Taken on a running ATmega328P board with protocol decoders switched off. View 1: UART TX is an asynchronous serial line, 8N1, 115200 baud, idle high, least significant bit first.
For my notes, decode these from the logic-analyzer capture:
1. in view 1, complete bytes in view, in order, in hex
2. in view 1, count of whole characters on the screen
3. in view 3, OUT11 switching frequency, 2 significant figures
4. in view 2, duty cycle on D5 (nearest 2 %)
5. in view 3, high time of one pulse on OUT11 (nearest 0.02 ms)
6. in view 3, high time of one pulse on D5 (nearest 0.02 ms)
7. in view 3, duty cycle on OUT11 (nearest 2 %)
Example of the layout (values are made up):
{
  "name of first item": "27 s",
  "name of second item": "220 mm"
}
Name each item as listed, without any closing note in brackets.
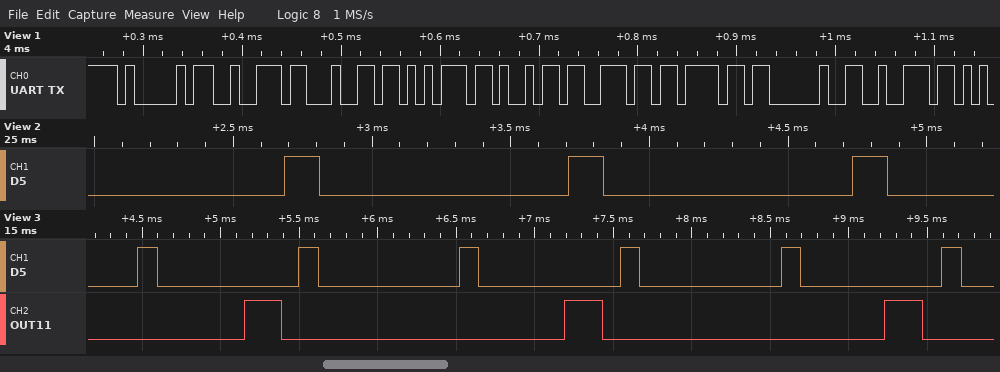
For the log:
{
  "in view 1, complete bytes in view, in order, in hex": "41 72 64 75 69 6E 6F 20 72",
  "in view 1, count of whole characters on the screen": "9",
  "in view 3, OUT11 switching frequency, 2 significant figures": "490 Hz",
  "in view 2, duty cycle on D5": "12 %",
  "in view 3, high time of one pulse on OUT11": "0.24 ms",
  "in view 3, high time of one pulse on D5": "0.12 ms",
  "in view 3, duty cycle on OUT11": "12 %"
}
